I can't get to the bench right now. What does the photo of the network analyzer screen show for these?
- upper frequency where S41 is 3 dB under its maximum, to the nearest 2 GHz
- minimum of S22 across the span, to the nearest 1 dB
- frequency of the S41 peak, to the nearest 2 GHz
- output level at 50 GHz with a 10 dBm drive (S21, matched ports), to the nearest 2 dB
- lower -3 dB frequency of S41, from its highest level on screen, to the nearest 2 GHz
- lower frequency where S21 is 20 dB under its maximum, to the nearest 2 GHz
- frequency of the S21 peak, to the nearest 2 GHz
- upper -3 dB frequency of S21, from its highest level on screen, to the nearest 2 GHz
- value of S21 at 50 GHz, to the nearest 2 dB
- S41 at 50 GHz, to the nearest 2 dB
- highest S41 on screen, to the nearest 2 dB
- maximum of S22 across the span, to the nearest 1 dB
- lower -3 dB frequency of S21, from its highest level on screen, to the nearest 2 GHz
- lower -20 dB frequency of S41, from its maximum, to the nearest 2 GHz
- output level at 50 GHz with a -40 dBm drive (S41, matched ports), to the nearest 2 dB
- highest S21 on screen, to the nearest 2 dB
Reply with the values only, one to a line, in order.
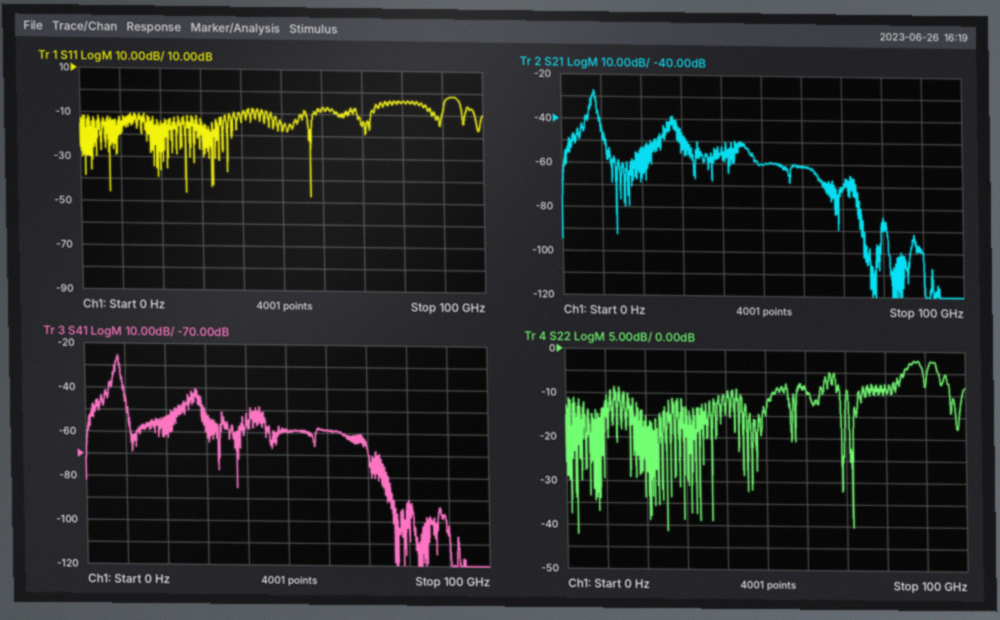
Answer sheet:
8 GHz
-42 dB
8 GHz
-50 dBm
8 GHz
4 GHz
8 GHz
8 GHz
-60 dB
-60 dB
-26 dB
-2 dB
8 GHz
4 GHz
-100 dBm
-28 dB
